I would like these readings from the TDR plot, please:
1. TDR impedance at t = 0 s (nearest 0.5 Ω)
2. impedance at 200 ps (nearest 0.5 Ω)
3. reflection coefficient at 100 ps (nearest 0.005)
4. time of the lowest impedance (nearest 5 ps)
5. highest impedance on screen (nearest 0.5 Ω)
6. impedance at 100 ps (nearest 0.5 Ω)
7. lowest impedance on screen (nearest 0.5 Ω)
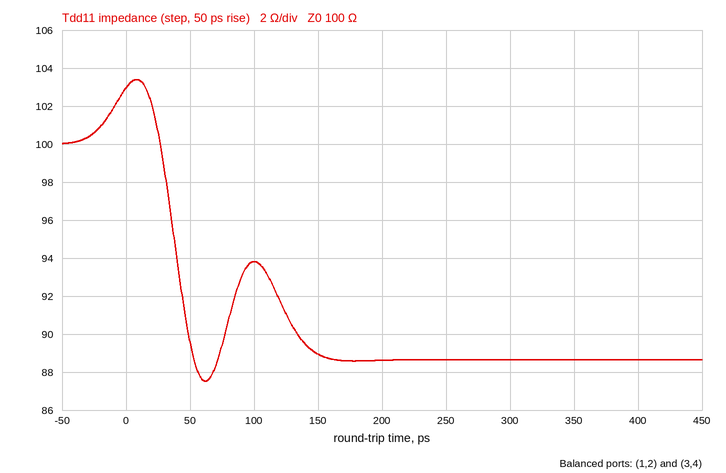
103.0 Ω
88.5 Ω
-0.030
60 ps
103.5 Ω
94.0 Ω
87.5 Ω
